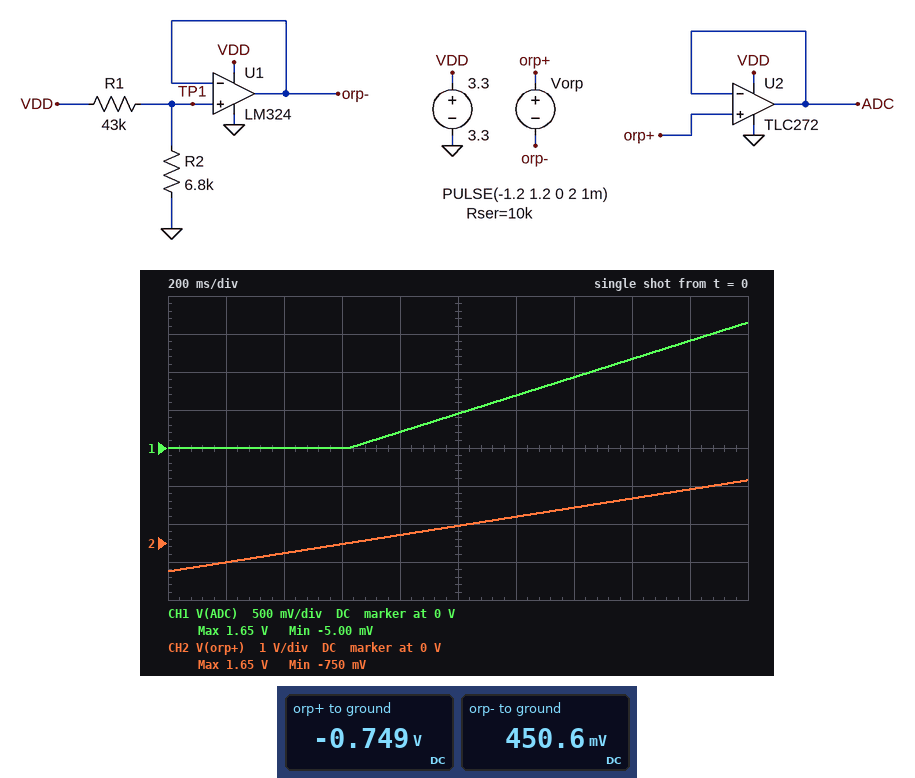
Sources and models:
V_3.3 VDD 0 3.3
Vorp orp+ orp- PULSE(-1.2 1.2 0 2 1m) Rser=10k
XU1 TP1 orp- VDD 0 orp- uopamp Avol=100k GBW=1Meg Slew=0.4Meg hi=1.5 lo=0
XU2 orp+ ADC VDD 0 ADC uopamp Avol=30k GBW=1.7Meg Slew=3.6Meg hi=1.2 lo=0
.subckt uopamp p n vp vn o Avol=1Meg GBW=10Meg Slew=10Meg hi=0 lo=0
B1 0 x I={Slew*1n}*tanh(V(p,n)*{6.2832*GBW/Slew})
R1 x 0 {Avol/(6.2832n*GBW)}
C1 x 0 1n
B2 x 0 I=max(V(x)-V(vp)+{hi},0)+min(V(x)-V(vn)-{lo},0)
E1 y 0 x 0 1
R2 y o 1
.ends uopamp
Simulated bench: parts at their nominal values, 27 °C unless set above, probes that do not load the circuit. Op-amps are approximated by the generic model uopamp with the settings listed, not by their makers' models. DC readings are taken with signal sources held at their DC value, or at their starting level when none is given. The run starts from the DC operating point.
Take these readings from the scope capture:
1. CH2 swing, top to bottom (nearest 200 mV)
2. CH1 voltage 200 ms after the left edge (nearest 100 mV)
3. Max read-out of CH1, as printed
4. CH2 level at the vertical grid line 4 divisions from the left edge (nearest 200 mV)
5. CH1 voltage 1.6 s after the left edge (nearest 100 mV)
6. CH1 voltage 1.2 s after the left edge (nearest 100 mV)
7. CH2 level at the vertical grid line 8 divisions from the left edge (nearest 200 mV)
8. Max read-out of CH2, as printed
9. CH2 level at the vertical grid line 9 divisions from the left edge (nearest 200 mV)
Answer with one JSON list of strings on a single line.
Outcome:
["2.4 V", "0 V", "1.65 V", "200 mV", "1.2 V", "700 mV", "1.2 V", "1.65 V", "1.4 V"]
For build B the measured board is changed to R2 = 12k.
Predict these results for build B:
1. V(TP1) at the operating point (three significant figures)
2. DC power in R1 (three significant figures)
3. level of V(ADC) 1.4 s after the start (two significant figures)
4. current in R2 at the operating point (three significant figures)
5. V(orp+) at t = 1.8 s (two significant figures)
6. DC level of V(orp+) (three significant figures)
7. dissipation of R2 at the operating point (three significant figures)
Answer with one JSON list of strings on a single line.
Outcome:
["720 mV", "155 µW", "1.2 V", "60.0 µA", "1.7 V", "-480 mV", "43.2 µW"]
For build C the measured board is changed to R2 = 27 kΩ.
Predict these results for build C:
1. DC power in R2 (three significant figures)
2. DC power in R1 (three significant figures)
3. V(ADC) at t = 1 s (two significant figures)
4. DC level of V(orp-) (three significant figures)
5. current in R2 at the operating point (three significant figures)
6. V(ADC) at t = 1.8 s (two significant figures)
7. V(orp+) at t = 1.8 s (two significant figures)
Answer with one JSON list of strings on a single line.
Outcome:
["60.0 µW", "95.6 µW", "1.3 V", "1.27 V", "47.1 µA", "2.1 V", "2.2 V"]
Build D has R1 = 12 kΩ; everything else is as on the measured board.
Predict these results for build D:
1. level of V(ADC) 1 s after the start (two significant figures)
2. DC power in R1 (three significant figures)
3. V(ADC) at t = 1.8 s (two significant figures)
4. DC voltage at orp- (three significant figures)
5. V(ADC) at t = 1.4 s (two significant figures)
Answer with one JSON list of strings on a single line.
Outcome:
["1.2 V", "370 µW", "2.1 V", "1.19 V", "1.7 V"]
